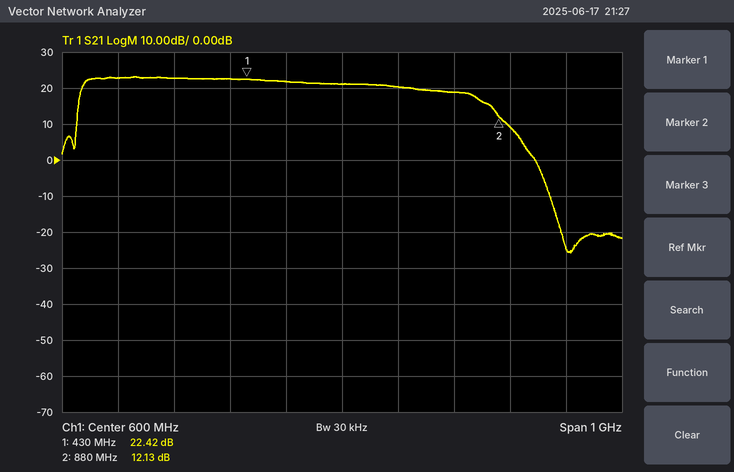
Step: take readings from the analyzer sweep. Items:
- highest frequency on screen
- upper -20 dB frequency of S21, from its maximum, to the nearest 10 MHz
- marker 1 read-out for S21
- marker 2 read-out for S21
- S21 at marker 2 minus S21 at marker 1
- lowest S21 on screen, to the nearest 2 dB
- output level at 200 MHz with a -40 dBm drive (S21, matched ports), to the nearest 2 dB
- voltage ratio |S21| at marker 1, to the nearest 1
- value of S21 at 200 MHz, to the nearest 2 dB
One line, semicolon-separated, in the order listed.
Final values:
1.1 GHz; 930 MHz; 22.42 dB; 12.13 dB; -10.29 dB; -26 dB; -18 dBm; 13; 22 dB
